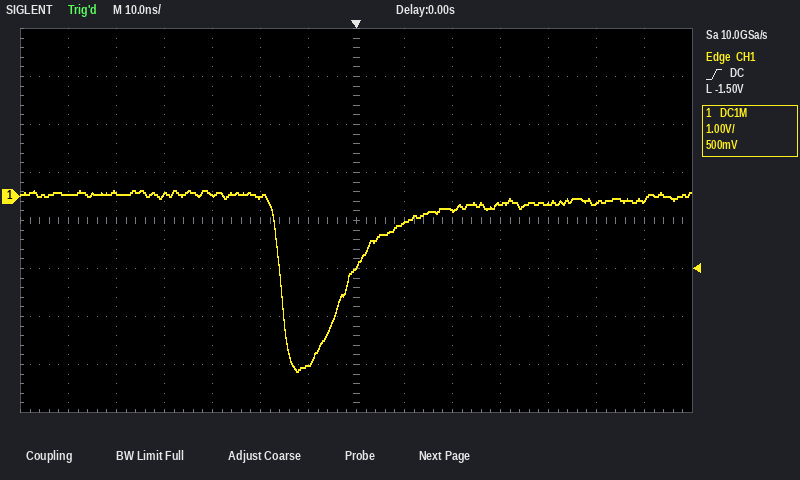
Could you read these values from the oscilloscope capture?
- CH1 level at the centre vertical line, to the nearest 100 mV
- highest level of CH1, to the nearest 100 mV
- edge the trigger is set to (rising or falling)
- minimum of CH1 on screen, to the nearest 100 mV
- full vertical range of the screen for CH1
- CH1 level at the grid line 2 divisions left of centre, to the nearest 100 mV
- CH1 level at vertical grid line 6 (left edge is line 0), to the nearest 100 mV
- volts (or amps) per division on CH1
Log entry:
-1.5 V
100 mV
rising
-3.6 V
8 V
0.0 V
-3.5 V
1 V
